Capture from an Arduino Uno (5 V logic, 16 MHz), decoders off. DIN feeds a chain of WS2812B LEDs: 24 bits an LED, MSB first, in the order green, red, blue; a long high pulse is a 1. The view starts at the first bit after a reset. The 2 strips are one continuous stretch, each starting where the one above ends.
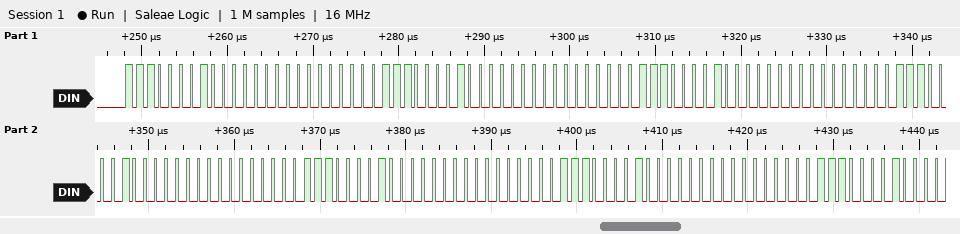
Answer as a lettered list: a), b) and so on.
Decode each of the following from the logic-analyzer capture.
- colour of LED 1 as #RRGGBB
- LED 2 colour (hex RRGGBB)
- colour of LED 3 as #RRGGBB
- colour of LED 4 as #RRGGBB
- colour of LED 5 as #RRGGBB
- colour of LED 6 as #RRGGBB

a) #00E100
b) #00E100
c) #00E100
d) #00E100
e) #00E100
f) #00E100
